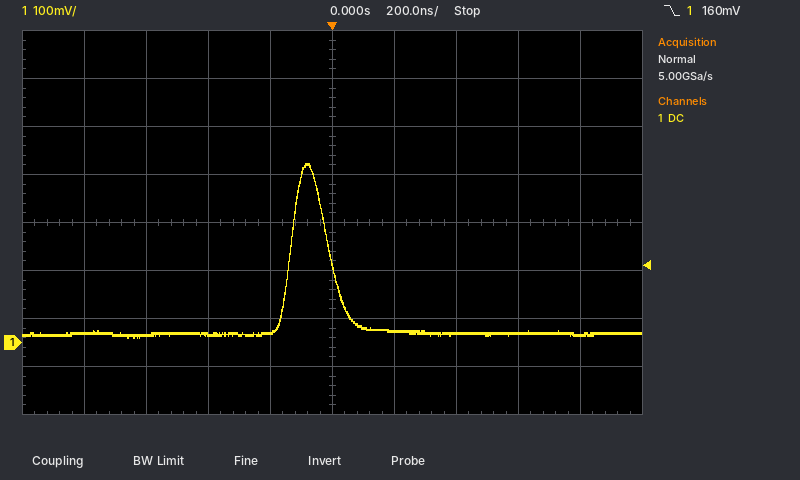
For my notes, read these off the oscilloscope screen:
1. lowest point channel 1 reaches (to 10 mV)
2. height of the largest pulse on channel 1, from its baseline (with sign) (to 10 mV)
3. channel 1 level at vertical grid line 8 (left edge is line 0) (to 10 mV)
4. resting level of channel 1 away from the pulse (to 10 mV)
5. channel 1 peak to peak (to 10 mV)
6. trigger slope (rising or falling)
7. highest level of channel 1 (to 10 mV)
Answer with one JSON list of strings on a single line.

["10 mV", "+350 mV", "20 mV", "20 mV", "360 mV", "falling", "370 mV"]
